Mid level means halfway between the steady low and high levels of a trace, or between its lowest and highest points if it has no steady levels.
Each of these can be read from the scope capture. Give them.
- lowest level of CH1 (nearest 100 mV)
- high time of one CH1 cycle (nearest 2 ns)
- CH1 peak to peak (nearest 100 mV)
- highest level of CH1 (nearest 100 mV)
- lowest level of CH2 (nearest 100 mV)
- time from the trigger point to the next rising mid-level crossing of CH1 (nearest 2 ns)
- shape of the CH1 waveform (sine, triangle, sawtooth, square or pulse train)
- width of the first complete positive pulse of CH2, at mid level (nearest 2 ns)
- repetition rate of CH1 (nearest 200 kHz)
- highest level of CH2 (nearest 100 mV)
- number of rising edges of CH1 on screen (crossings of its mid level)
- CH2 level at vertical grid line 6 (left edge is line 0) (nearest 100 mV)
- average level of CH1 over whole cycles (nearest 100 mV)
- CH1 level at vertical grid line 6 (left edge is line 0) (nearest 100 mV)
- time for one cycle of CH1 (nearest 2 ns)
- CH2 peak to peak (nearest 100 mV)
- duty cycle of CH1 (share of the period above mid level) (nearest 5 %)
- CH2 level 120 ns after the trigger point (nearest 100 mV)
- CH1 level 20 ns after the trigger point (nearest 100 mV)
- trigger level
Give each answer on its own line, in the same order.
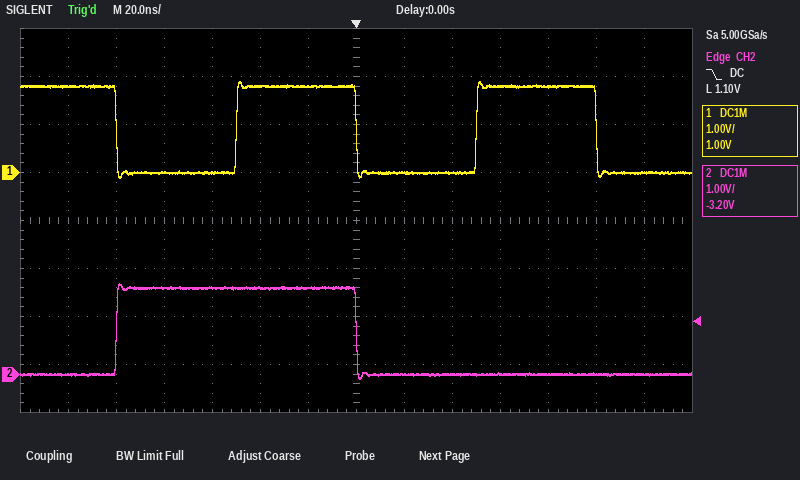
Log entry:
-100 mV
50 ns
2.0 V
1.9 V
-100 mV
50 ns
square
100 ns
10.0 MHz
1.9 V
2
1.8 V
900 mV
1.8 V
100 ns
2.0 V
50 %
0.0 V
0.0 V
1.10 V
